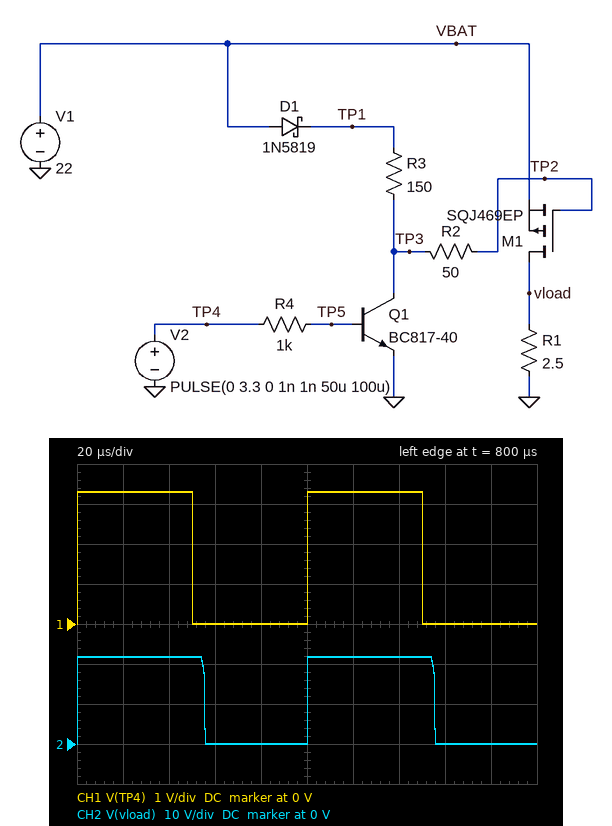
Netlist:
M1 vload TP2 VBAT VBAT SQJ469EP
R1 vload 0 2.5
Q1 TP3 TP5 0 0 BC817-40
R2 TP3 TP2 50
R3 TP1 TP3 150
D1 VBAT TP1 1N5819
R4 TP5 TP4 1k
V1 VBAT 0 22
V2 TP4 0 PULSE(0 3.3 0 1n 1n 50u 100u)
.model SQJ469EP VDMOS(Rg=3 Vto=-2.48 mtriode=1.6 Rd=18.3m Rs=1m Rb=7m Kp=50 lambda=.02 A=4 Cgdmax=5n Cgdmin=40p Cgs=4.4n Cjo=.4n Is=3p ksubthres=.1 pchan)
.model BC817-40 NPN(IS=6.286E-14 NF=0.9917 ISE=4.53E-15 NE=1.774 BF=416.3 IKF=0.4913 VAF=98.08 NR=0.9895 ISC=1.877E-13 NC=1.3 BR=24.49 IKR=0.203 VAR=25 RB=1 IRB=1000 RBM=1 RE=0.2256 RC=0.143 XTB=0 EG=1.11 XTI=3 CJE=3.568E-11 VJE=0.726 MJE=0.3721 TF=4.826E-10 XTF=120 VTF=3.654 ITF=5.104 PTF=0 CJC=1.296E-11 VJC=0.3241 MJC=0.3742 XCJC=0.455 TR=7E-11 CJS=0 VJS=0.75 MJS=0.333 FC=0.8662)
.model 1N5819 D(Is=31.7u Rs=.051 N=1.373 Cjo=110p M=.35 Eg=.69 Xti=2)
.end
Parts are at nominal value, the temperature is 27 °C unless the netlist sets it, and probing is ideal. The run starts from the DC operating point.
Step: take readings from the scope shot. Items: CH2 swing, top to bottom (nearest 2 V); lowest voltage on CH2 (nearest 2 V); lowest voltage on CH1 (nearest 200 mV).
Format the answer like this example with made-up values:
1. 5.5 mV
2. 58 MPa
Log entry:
1. 22 V
2. 0 V
3. 0 V
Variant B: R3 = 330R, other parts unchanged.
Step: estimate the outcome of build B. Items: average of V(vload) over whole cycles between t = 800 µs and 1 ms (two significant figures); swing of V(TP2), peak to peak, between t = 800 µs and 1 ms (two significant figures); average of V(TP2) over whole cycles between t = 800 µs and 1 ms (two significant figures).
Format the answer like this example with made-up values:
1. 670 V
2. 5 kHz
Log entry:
1. 13 V
2. 22 V
3. 10 V
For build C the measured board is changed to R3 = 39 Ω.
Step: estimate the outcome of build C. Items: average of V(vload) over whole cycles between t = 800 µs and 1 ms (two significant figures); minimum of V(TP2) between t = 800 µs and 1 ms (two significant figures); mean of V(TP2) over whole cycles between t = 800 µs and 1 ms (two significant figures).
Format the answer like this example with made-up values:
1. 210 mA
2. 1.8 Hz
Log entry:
1. 11 V
2. 2.5 V
3. 12 V
